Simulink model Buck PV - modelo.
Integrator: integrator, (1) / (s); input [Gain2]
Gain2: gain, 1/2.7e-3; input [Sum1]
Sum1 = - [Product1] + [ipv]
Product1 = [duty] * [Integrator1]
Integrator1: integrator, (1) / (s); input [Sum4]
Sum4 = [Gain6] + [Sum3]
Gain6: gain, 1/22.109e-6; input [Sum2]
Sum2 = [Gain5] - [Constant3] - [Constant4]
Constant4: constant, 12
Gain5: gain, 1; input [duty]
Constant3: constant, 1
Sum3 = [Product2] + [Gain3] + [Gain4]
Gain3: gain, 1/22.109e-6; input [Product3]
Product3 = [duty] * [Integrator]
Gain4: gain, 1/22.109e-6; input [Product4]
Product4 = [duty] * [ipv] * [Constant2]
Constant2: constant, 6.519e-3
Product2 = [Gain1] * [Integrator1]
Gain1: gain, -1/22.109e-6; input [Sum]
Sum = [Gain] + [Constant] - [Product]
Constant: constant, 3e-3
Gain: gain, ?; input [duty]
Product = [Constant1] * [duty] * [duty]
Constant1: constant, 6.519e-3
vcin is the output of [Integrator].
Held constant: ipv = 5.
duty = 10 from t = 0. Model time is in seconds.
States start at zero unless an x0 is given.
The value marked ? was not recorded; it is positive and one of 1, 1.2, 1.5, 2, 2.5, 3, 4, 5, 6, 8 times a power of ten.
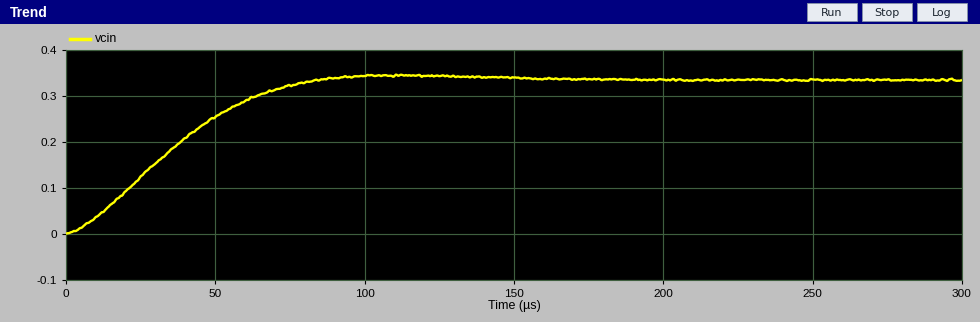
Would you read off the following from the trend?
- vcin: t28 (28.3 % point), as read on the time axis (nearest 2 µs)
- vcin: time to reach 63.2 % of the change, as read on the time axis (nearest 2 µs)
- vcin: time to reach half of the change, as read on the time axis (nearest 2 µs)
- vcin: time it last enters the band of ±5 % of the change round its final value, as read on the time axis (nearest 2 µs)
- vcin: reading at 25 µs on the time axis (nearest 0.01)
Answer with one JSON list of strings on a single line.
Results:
["20 µs", "40 µs", "32 µs", "72 µs", "0.12"]
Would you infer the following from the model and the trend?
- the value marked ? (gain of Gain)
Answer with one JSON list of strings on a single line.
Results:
["0.2"]
